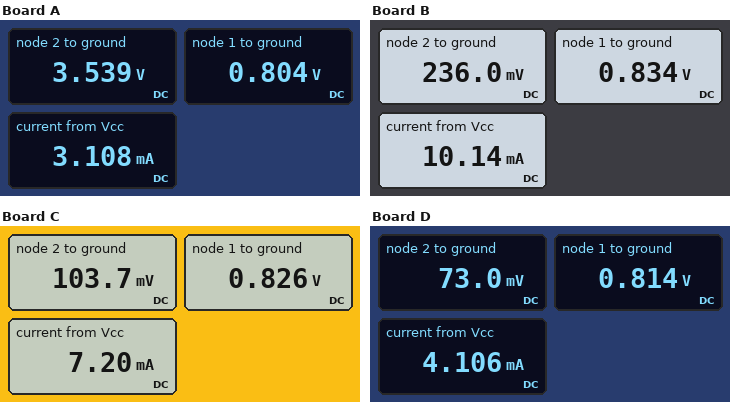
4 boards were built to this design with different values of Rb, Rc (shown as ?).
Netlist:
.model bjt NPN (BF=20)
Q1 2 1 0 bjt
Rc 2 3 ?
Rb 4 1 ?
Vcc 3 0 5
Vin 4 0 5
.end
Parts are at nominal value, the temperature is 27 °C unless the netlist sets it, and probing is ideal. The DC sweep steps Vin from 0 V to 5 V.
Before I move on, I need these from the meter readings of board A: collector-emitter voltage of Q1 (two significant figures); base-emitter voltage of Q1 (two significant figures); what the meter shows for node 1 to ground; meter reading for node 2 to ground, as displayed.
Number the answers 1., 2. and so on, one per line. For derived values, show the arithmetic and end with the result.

1. 3.539 V = 3.5 V
2. 804 mV = 800 mV
3. 0.804 V
4. 3.539 V
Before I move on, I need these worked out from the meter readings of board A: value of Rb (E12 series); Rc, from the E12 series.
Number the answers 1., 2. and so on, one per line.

1. 27 kΩ
2. 470 Ω
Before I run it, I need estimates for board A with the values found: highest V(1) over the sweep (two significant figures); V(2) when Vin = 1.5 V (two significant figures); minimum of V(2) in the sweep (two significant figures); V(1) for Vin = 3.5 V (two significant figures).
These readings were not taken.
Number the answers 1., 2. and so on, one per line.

1. 800 mV
2. 4.7 V
3. 3.5 V
4. 790 mV
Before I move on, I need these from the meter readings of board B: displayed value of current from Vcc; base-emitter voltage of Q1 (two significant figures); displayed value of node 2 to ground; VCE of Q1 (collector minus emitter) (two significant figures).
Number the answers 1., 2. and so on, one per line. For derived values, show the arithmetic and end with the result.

1. 10.14 mA
2. 834 mV = 830 mV
3. 236.0 mV
4. 236 mV = 240 mV
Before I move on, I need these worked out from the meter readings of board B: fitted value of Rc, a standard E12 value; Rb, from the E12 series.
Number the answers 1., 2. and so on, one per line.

1. 470 Ω
2. 8.2 kΩ
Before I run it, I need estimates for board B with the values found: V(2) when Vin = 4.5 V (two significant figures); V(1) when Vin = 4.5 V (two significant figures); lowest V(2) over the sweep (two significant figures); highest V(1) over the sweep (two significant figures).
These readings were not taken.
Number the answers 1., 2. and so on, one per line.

1. 790 mV
2. 830 mV
3. 240 mV
4. 830 mV
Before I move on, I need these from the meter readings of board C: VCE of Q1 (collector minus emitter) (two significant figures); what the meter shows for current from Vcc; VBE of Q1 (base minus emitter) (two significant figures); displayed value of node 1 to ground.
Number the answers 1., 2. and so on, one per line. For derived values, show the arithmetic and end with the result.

1. 103.7 mV = 100 mV
2. 7.20 mA
3. 826 mV = 830 mV
4. 0.826 V
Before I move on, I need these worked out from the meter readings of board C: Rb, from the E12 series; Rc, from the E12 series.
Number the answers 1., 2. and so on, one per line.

1. 8.2 kΩ
2. 680 Ω
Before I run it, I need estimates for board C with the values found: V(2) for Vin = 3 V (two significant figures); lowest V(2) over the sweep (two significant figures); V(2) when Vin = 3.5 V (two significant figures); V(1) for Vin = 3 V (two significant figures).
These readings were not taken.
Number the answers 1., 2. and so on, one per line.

1. 1.4 V
2. 100 mV
3. 560 mV
4. 820 mV
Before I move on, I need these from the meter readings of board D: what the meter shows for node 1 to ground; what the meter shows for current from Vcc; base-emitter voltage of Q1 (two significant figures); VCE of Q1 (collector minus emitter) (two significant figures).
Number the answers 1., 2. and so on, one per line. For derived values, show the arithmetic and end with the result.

1. 0.814 V
2. 4.106 mA
3. 814 mV = 810 mV
4. 73 mV = 73 mV
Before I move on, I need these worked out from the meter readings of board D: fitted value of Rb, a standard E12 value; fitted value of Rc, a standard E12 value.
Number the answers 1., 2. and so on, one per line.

1. 8.2 kΩ
2. 1.2 kΩ
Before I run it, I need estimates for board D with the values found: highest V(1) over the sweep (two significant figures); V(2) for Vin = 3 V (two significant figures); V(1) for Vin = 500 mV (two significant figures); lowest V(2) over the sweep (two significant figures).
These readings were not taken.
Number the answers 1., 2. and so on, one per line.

1. 810 mV
2. 110 mV
3. 500 mV
4. 73 mV
